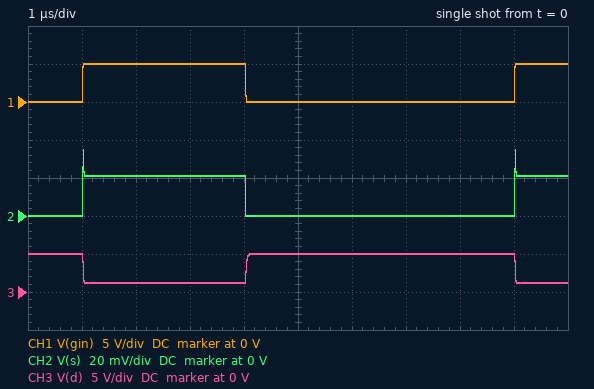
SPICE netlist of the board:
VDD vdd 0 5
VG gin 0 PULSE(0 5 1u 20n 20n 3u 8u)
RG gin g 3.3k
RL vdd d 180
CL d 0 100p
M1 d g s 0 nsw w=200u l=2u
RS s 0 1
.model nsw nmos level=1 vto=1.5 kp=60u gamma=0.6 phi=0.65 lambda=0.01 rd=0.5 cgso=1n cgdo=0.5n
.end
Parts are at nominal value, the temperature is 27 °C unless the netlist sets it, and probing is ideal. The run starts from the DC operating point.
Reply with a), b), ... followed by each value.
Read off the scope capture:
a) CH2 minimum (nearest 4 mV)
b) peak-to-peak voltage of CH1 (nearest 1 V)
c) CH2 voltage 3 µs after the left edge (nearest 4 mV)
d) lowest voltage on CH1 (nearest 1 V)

a) 0 V
b) 5 V
c) 20 mV
d) 0 V
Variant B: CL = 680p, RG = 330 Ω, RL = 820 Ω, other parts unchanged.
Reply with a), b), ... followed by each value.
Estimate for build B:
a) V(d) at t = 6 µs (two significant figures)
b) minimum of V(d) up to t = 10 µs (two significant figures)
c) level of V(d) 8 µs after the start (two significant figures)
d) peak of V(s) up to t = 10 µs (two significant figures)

a) 4.9 V
b) 290 mV
c) 5.0 V
d) 37 mV
